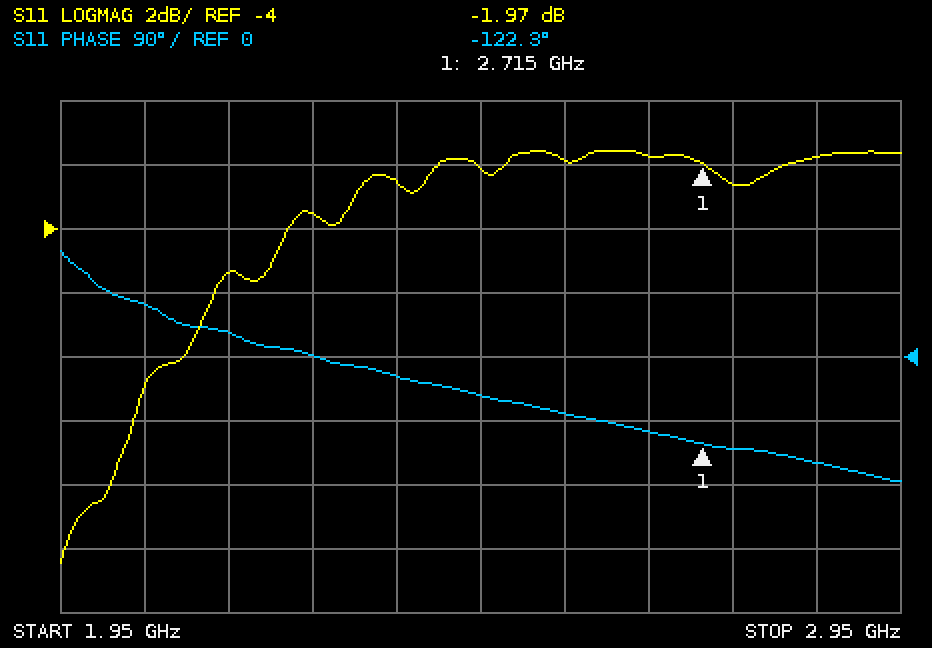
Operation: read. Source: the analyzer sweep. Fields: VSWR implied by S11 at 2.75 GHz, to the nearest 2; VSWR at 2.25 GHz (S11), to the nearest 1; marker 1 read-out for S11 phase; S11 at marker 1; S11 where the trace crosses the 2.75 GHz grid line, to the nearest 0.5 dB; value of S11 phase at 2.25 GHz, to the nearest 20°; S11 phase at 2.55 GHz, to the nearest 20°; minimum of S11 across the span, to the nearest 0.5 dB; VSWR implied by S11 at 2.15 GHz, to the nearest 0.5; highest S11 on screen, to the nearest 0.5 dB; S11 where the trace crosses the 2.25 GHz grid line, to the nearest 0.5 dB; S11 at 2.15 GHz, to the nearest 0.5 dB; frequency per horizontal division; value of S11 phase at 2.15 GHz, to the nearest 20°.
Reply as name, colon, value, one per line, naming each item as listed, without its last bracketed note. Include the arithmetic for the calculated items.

VSWR implied by S11 at 2.75 GHz, to the nearest 2: |Γ| = 10^(-2.5/20) = 0.7499; VSWR = (1 + 0.7499)/(1 − 0.7499) ≈ 7.00, so 6 to the nearest 2
VSWR at 2.25 GHz (S11), to the nearest 1: |Γ| = 10^(-3.5/20) = 0.6683; VSWR = (1 + 0.6683)/(1 − 0.6683) ≈ 5
marker 1 read-out for S11 phase: -122.3°
S11 at marker 1: -1.97 dB
S11 where the trace crosses the 2.75 GHz grid line, to the nearest 0.5 dB: -2.5 dB
value of S11 phase at 2.25 GHz, to the nearest 20°: 0°
S11 phase at 2.55 GHz, to the nearest 20°: -80°
minimum of S11 across the span, to the nearest 0.5 dB: -14.5 dB
VSWR implied by S11 at 2.15 GHz, to the nearest 0.5: |Γ| = 10^(-5.5/20) = 0.5309; VSWR = (1 + 0.5309)/(1 − 0.5309) ≈ 3.26, so 3.5 to the nearest 0.5
highest S11 on screen, to the nearest 0.5 dB: -1.5 dB
S11 where the trace crosses the 2.25 GHz grid line, to the nearest 0.5 dB: -3.5 dB
S11 at 2.15 GHz, to the nearest 0.5 dB: -5.5 dB
frequency per horizontal division: 100 MHz
value of S11 phase at 2.15 GHz, to the nearest 20°: 40°
